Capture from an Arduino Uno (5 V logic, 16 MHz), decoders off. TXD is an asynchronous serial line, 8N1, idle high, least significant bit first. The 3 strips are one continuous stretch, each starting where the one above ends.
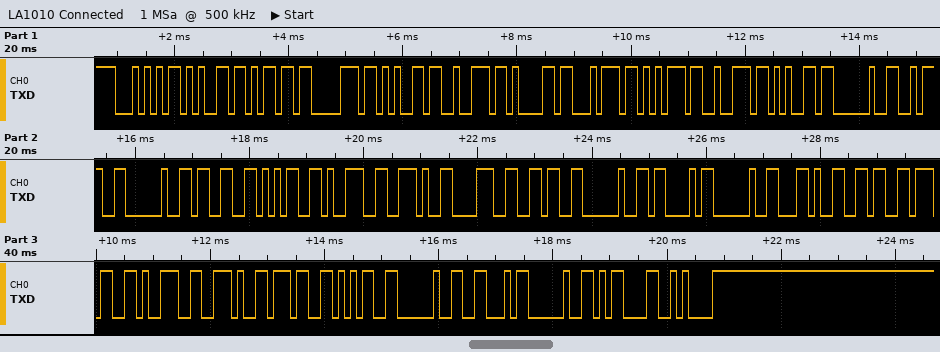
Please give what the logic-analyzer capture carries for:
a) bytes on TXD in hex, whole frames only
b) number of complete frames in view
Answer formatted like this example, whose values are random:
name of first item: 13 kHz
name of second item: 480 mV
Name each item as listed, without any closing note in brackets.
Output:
bytes on TXD in hex, whole frames only: 0x54 0x65 0x6D 0x70 0x65 0x72 0x61 0x74 0x75 0x72 0x65 0x20 0x3A 0x20 0x33 0x35 0x39 0x2E 0x38 0x36 0x20 0x43 0x20 0x2C 0x36 0x37 0x39 0x2E 0x37 0x35 0x20 0x46 0x20 0x0D 0x0A
number of complete frames in view: 35
